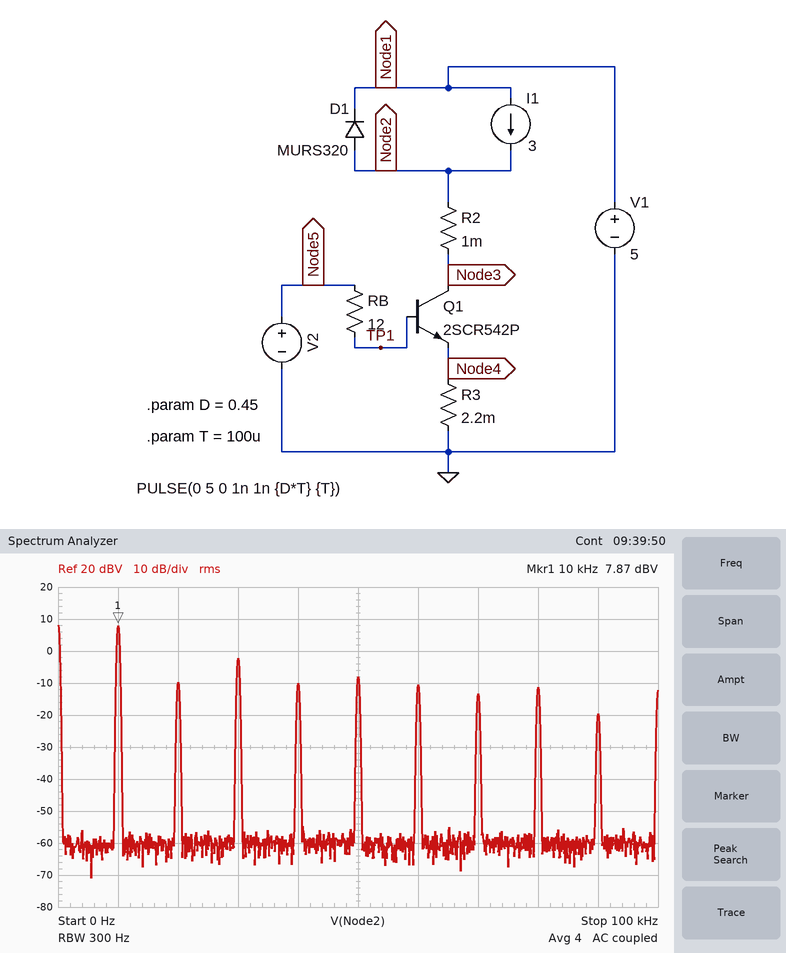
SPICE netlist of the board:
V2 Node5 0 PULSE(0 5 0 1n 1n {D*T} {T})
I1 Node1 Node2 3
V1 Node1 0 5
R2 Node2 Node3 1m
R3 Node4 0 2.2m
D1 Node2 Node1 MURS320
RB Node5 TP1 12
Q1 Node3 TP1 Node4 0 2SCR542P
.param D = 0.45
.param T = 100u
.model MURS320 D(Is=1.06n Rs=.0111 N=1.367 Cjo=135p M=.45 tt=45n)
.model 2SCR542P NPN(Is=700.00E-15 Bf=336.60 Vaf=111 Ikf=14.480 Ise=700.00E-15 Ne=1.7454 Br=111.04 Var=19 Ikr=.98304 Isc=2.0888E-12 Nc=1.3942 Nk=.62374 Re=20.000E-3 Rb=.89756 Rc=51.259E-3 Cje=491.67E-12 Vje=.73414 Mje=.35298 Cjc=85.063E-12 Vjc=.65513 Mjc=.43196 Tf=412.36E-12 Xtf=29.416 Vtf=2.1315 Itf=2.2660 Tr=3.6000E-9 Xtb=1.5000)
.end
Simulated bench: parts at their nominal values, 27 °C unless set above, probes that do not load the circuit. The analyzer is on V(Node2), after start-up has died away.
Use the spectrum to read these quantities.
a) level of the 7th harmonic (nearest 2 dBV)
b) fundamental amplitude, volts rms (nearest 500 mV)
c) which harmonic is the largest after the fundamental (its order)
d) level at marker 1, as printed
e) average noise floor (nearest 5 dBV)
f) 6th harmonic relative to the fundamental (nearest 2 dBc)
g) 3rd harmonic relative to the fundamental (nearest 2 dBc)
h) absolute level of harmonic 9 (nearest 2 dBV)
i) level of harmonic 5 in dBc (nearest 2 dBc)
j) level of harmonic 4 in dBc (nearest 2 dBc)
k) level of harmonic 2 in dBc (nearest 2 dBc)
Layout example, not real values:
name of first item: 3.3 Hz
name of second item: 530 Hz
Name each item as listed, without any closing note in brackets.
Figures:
level of the 7th harmonic: -14 dBV
fundamental amplitude, volts rms: 2.5 V
which harmonic is the largest after the fundamental: 3
level at marker 1, as printed: 7.87 dBV
average noise floor: -60 dBV
6th harmonic relative to the fundamental: -18 dBc
3rd harmonic relative to the fundamental: -10 dBc
absolute level of harmonic 9: -20 dBV
level of harmonic 5 in dBc: -16 dBc
level of harmonic 4 in dBc: -18 dBc
level of harmonic 2 in dBc: -18 dBc
